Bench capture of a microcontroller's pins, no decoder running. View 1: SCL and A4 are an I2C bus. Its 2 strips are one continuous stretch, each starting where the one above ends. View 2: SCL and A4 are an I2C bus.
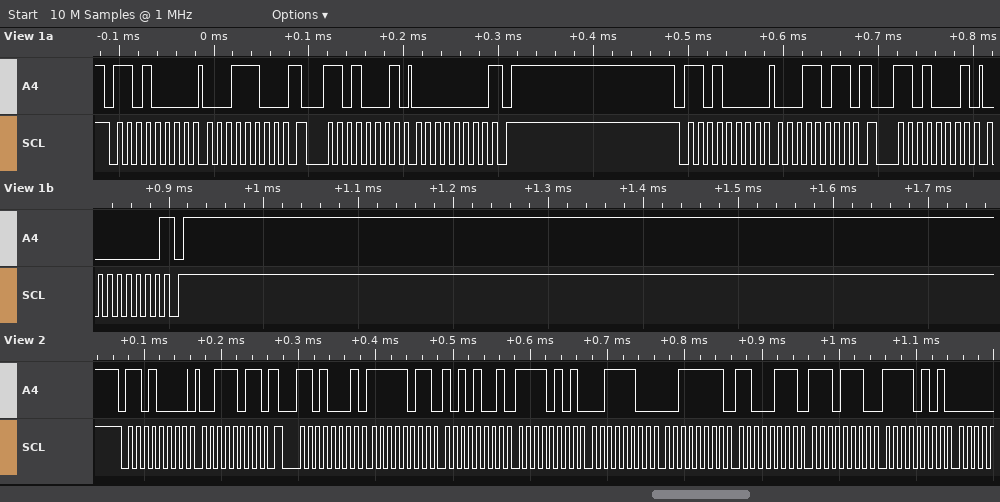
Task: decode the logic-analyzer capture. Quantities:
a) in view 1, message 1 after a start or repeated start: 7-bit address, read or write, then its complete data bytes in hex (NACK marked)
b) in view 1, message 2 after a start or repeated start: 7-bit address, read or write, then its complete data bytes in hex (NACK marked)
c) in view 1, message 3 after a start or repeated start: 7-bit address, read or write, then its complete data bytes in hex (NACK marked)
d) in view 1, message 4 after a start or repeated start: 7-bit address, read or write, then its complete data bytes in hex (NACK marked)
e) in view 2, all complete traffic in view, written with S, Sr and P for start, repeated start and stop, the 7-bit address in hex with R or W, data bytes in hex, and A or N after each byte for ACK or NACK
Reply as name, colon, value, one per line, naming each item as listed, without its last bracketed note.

in view 1, message 1 after a start or repeated start: 7-bit address, read or write, then its complete data bytes in hex: 0x68 write: 1C
in view 1, message 2 after a start or repeated start: 7-bit address, read or write, then its complete data bytes in hex: 0x68 read: 00 NACK
in view 1, message 3 after a start or repeated start: 7-bit address, read or write, then its complete data bytes in hex: 0x68 write: 1B
in view 1, message 4 after a start or repeated start: 7-bit address, read or write, then its complete data bytes in hex: 0x68 read: 00 NACK
in view 2, all complete traffic in view, written with S, Sr and P for start, repeated start and stop, the 7-bit address in hex with R or W, data bytes in hex, and A or N after each byte for ACK or NACK: S 68W A 3B A Sr 68R A FB A A9 A F5 A 3C A 3F A C7 A EE A F5 A
